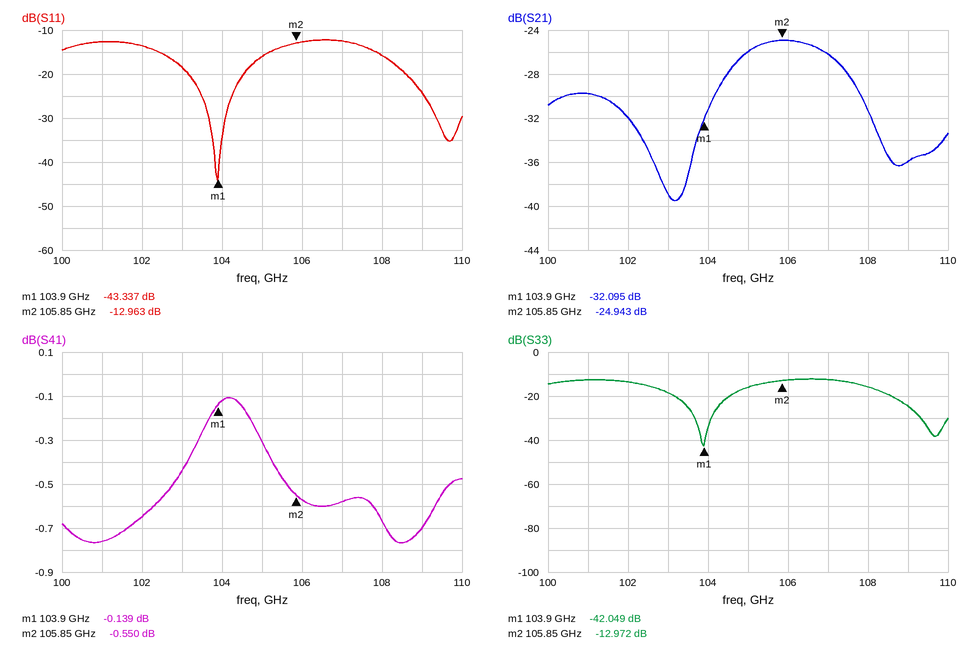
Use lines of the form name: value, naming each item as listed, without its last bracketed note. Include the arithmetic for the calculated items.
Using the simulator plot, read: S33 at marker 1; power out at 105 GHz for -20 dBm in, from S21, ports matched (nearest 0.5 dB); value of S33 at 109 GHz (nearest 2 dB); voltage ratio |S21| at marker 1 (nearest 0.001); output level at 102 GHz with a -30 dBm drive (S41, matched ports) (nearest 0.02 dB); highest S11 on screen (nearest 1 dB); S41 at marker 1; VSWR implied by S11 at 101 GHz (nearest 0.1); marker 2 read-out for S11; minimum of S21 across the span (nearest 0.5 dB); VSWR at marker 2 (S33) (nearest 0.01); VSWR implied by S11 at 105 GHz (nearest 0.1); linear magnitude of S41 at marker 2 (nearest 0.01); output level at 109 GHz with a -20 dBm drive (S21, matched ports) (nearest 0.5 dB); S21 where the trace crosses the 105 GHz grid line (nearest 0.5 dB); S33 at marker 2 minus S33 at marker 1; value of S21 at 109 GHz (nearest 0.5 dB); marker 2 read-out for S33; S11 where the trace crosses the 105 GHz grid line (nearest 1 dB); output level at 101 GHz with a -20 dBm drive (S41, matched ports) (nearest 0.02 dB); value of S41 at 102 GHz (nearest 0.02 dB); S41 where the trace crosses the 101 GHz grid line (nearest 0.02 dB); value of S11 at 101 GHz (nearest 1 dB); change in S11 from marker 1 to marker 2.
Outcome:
S33 at marker 1: -42.049 dB
power out at 105 GHz for -20 dBm in, from S21, ports matched: -20 dBm + (-26.0 dB) = -46.0 dBm
value of S33 at 109 GHz: -24 dB
voltage ratio |S21| at marker 1: 10^(-32.095/20) ≈ 0.025
output level at 102 GHz with a -30 dBm drive (S41, matched ports): -30 dBm + (-0.64 dB) = -30.64 dBm
highest S11 on screen: -12 dB
S41 at marker 1: -0.139 dB
VSWR implied by S11 at 101 GHz: |Γ| = 10^(-13/20) = 0.2239; VSWR = (1 + 0.2239)/(1 − 0.2239) ≈ 1.6
marker 2 read-out for S11: -12.963 dB
minimum of S21 across the span: -39.5 dB
VSWR at marker 2 (S33): (1 + 0.2246)/(1 − 0.2246) ≈ 1.58
VSWR implied by S11 at 105 GHz: |Γ| = 10^(-16/20) = 0.1585; VSWR = (1 + 0.1585)/(1 − 0.1585) ≈ 1.4
linear magnitude of S41 at marker 2: 10^(-0.55/20) ≈ 0.94
output level at 109 GHz with a -20 dBm drive (S21, matched ports): -20 dBm + (-36.0 dB) = -56.0 dBm
S21 where the trace crosses the 105 GHz grid line: -26.0 dB
S33 at marker 2 minus S33 at marker 1: -12.972 − (-42.049) = 29.077 dB
value of S21 at 109 GHz: -36.0 dB
marker 2 read-out for S33: -12.972 dB
S11 where the trace crosses the 105 GHz grid line: -16 dB
output level at 101 GHz with a -20 dBm drive (S41, matched ports): -20 dBm + (-0.76 dB) = -20.76 dBm
value of S41 at 102 GHz: -0.64 dB
S41 where the trace crosses the 101 GHz grid line: -0.76 dB
value of S11 at 101 GHz: -13 dB
change in S11 from marker 1 to marker 2: -12.963 − (-43.337) = 30.374 dB
